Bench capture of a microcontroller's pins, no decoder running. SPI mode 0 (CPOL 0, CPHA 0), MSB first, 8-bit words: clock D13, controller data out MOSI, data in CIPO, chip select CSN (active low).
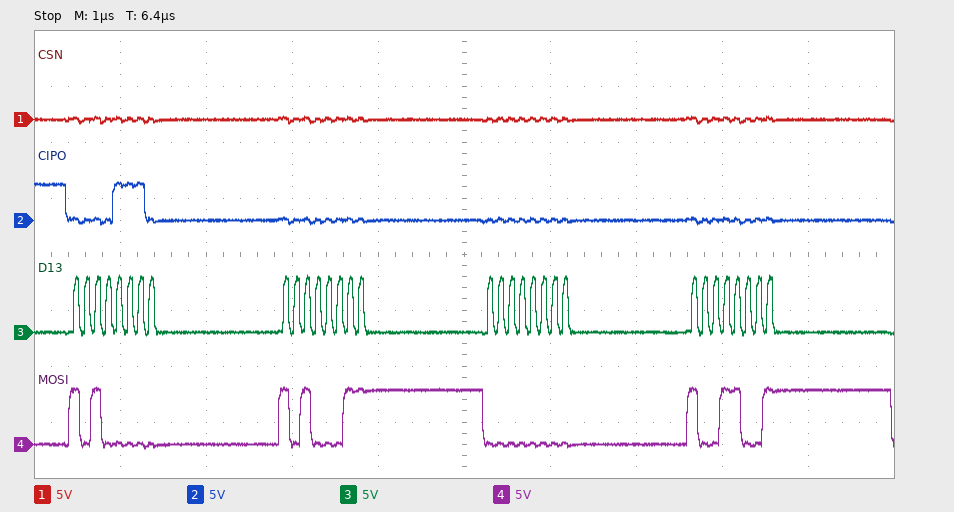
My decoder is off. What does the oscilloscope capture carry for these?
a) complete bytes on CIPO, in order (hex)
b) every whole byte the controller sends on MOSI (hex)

0E 00 00 00
A0 A3 00 99
